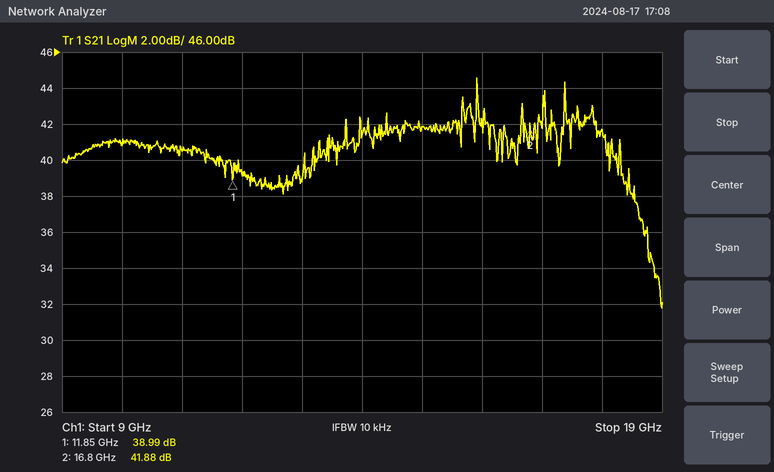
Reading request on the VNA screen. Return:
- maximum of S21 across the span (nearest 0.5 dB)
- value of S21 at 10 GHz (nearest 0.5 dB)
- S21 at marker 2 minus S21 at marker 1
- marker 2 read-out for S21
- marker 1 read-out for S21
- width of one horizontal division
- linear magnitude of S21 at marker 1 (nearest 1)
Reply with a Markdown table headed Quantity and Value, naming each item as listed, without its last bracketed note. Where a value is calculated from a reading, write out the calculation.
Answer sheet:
| Quantity | Value |
|---|---|
| maximum of S21 across the span | 44.5 dB |
| value of S21 at 10 GHz | 41.0 dB |
| S21 at marker 2 minus S21 at marker 1 | 41.88 − (38.99) = 2.89 dB |
| marker 2 read-out for S21 | 41.88 dB |
| marker 1 read-out for S21 | 38.99 dB |
| width of one horizontal division | 1 GHz |
| linear magnitude of S21 at marker 1 | 10^(38.99/20) ≈ 89 |
